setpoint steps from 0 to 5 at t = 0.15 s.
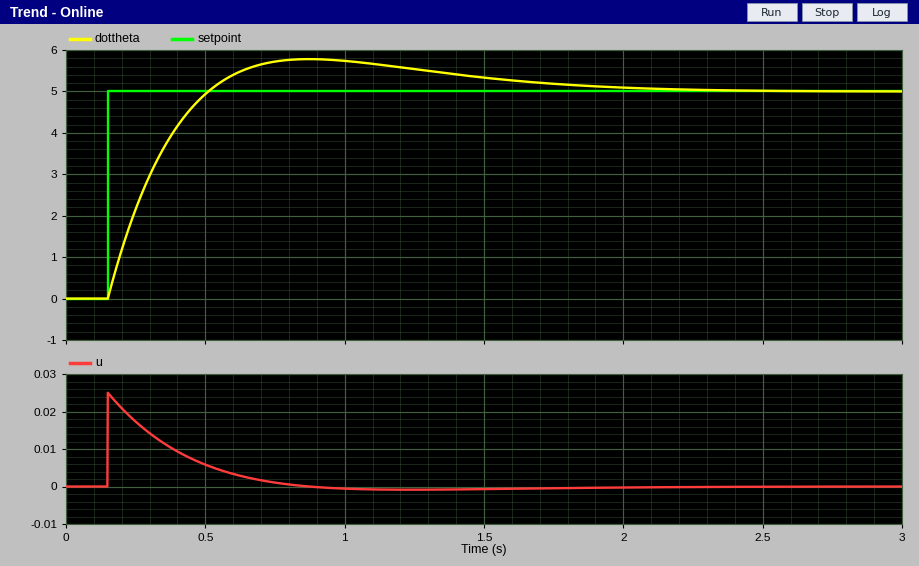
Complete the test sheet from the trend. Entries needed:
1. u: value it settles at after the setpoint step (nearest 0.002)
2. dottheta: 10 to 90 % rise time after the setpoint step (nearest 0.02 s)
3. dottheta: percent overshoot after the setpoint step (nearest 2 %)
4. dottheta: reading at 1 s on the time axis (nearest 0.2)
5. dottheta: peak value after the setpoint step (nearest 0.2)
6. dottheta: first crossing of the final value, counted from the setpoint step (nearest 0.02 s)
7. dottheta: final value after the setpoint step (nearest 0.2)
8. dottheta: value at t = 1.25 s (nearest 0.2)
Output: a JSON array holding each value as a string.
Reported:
["0.000", "0.26 s", "16 %", "5.8", "5.8", "0.36 s", "5.0", "5.6"]
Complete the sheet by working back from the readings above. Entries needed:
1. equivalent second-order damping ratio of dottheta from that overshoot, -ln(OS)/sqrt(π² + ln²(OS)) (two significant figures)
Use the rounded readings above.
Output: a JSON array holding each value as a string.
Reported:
["0.50"]
